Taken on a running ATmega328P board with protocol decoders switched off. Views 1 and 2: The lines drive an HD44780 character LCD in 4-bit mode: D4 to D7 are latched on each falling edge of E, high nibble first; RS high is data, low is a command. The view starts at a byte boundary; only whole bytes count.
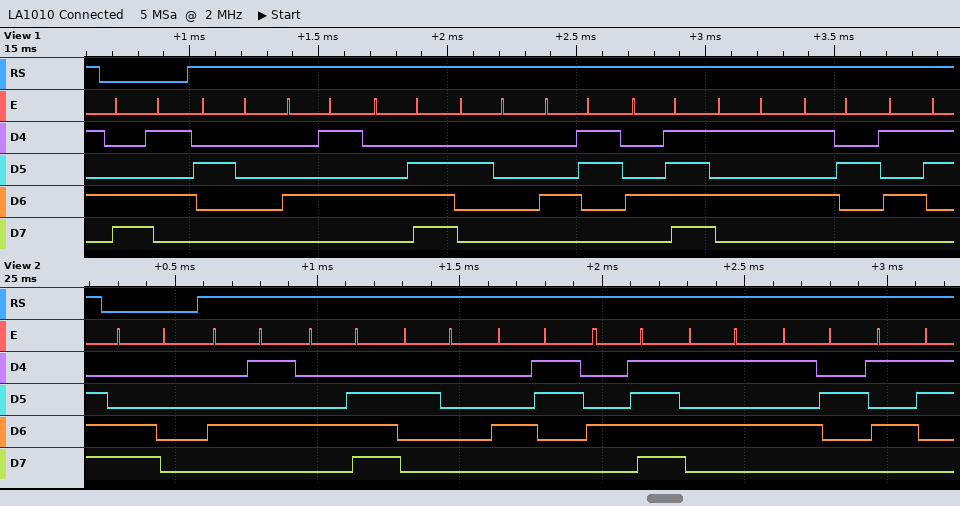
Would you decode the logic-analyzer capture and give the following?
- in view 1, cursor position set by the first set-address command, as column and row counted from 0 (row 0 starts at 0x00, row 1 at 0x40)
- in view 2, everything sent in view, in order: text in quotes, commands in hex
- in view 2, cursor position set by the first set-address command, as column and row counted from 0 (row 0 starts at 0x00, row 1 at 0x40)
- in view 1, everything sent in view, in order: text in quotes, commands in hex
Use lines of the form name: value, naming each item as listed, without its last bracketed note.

in view 1, cursor position set by the first set-address command, as column and row counted from 0: column 5, row 1
in view 2, everything sent in view, in order: text in quotes, commands in hex: 0xC0 "EN COURS"
in view 2, cursor position set by the first set-address command, as column and row counted from 0: column 0, row 1
in view 1, everything sent in view, in order: text in quotes, commands in hex: 0xC5 " EN COURS"
